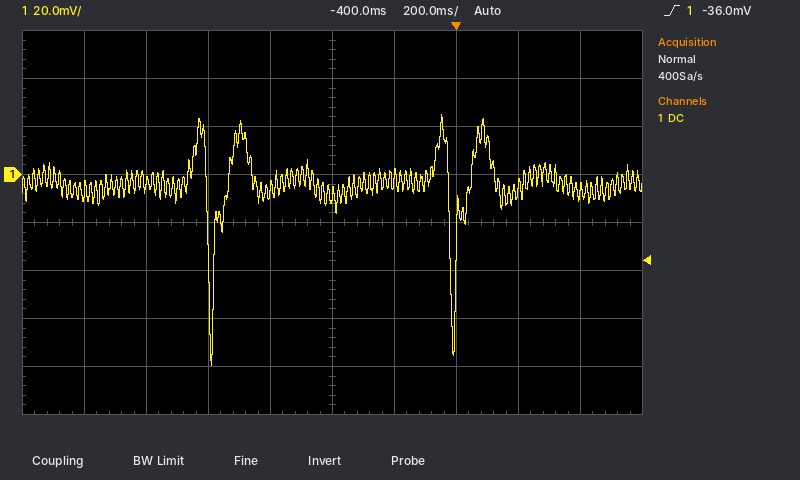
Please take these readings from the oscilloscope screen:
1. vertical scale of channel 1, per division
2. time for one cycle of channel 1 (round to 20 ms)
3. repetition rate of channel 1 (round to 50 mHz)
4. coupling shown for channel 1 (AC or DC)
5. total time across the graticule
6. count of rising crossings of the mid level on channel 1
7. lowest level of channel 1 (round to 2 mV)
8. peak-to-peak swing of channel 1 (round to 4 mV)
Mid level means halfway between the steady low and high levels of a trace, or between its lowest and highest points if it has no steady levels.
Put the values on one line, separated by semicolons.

20 mV; 780 ms; 1.30 Hz; DC; 2 s; 2; -80 mV; 104 mV
